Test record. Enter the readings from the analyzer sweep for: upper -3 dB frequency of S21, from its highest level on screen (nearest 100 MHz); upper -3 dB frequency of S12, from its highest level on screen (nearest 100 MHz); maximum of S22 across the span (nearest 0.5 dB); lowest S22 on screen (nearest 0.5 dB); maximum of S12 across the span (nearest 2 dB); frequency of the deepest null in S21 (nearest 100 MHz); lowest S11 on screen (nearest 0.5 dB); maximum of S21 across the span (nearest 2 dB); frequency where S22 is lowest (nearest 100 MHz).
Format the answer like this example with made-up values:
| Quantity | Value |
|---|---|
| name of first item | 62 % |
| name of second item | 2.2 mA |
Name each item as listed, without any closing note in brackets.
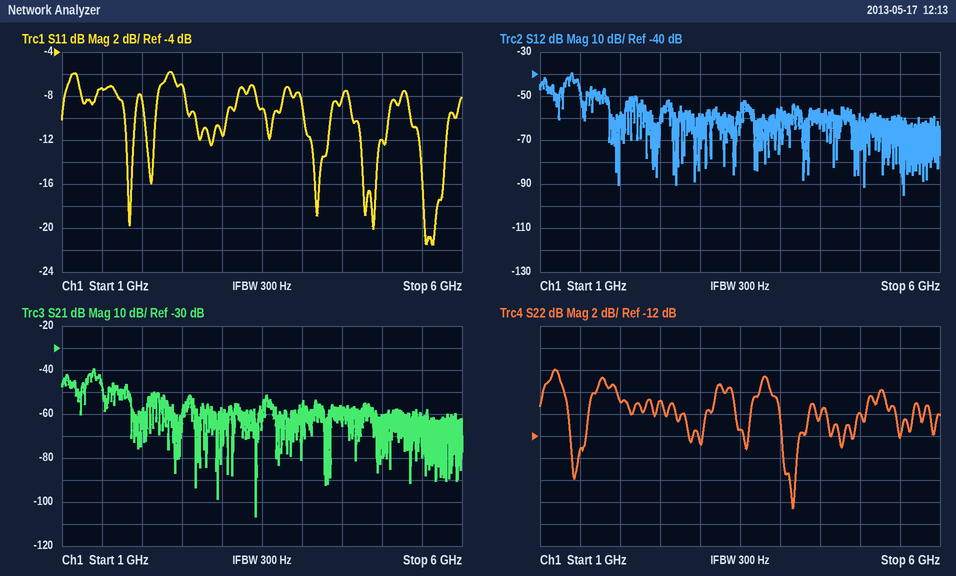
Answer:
| Quantity | Value |
|---|---|
| upper -3 dB frequency of S21, from its highest level on screen | 1.4 GHz |
| upper -3 dB frequency of S12, from its highest level on screen | 1.4 GHz |
| maximum of S22 across the span | -6.0 dB |
| lowest S22 on screen | -18.5 dB |
| maximum of S12 across the span | -40 dB |
| frequency of the deepest null in S21 | 3.4 GHz |
| lowest S11 on screen | -21.5 dB |
| maximum of S21 across the span | -40 dB |
| frequency where S22 is lowest | 4.2 GHz |
